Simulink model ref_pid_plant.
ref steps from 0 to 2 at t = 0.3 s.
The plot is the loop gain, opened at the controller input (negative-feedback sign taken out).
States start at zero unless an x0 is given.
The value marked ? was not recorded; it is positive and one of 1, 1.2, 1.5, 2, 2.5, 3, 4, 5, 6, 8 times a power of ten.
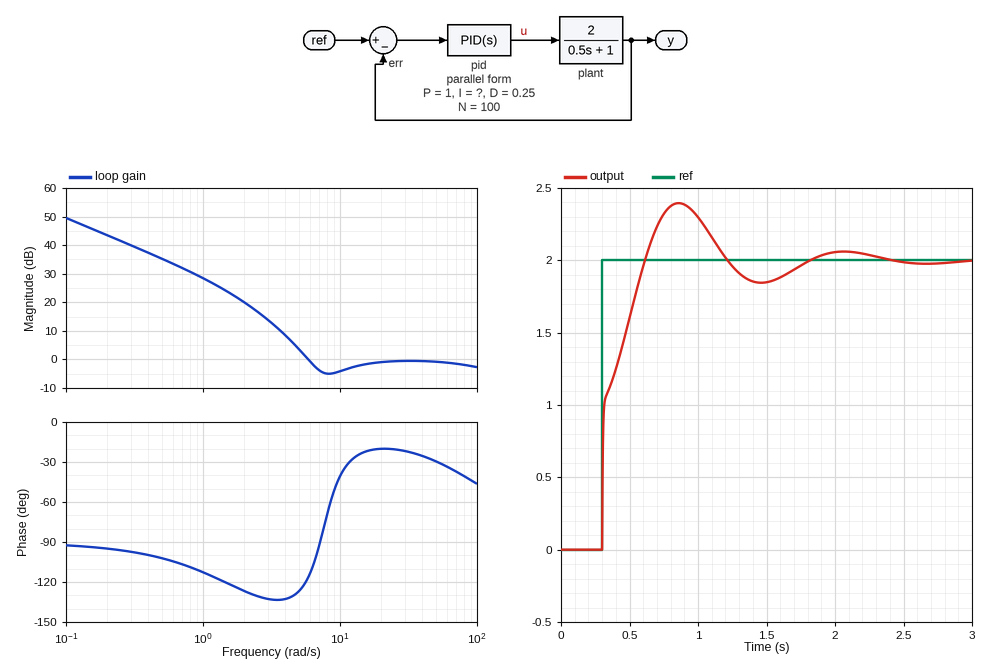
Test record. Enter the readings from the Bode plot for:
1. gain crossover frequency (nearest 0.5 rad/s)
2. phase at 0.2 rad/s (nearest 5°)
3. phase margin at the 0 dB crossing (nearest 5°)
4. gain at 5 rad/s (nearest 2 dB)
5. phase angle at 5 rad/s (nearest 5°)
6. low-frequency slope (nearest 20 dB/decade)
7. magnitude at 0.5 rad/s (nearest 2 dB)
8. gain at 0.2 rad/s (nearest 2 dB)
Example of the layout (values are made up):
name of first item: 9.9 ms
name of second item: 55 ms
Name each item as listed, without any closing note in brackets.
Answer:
gain crossover frequency: 6.0 rad/s
phase at 0.2 rad/s: -95°
phase margin at the 0 dB crossing: 65°
gain at 5 rad/s: 4 dB
phase angle at 5 rad/s: -125°
low-frequency slope: -20 dB/decade
magnitude at 0.5 rad/s: 36 dB
gain at 0.2 rad/s: 44 dB
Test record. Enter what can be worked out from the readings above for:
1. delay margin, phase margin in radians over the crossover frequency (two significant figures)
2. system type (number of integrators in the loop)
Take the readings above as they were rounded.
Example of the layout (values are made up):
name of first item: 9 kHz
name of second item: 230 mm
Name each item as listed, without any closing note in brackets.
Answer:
delay margin, phase margin in radians over the crossover frequency: 0.19 s
system type: 1
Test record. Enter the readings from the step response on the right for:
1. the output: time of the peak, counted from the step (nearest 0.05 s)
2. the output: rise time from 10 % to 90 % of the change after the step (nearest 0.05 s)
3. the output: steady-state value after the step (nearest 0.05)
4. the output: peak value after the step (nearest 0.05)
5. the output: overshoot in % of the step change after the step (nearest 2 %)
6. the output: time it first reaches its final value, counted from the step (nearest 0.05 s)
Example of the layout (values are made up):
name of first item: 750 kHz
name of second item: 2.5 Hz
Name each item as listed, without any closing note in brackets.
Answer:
the output: time of the peak, counted from the step: 0.55 s
the output: rise time from 10 % to 90 % of the change after the step: 0.25 s
the output: steady-state value after the step: 2.00
the output: peak value after the step: 2.40
the output: overshoot in % of the step change after the step: 20 %
the output: time it first reaches its final value, counted from the step: 0.30 s
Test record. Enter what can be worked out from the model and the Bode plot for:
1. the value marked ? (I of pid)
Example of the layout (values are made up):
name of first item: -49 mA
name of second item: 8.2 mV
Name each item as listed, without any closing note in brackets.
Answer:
the value marked ?: 15
